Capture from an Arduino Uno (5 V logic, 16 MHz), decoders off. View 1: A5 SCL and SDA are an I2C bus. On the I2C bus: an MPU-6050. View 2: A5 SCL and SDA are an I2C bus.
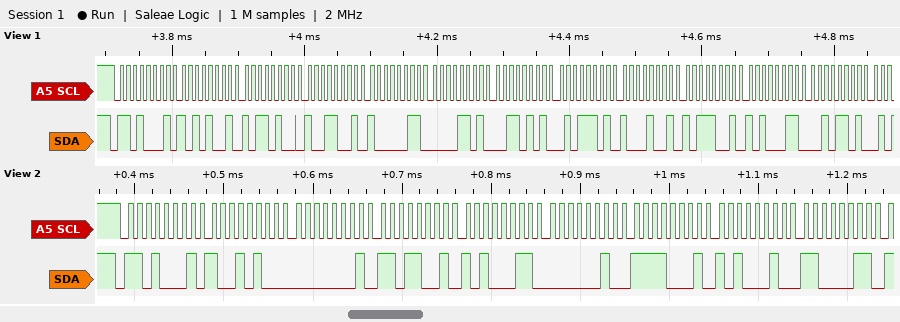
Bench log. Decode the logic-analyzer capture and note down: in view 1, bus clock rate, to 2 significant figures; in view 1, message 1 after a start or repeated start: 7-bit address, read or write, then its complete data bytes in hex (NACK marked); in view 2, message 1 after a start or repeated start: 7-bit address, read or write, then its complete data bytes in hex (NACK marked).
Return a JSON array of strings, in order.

["100 kHz", "0x68 read: A9 B4 99 83 0D 35 5D 89 B9 A3 2D", "0x68 read: 94 01 D9 A3 02 F1 A2 C3"]
